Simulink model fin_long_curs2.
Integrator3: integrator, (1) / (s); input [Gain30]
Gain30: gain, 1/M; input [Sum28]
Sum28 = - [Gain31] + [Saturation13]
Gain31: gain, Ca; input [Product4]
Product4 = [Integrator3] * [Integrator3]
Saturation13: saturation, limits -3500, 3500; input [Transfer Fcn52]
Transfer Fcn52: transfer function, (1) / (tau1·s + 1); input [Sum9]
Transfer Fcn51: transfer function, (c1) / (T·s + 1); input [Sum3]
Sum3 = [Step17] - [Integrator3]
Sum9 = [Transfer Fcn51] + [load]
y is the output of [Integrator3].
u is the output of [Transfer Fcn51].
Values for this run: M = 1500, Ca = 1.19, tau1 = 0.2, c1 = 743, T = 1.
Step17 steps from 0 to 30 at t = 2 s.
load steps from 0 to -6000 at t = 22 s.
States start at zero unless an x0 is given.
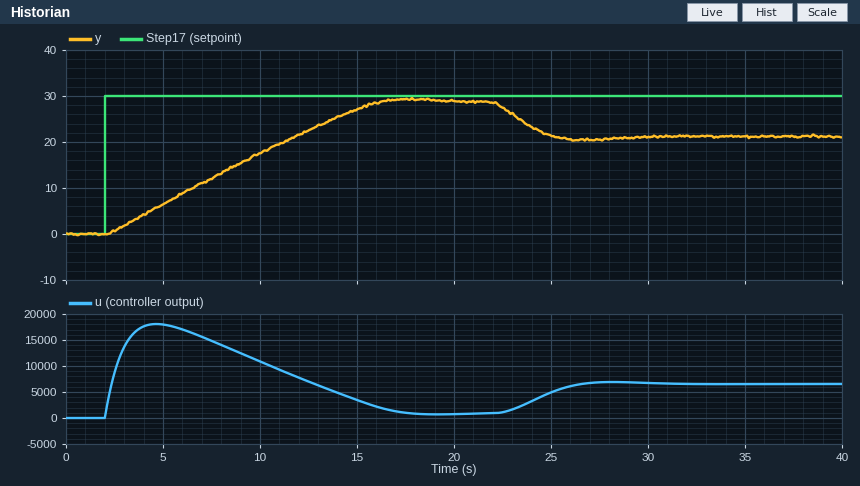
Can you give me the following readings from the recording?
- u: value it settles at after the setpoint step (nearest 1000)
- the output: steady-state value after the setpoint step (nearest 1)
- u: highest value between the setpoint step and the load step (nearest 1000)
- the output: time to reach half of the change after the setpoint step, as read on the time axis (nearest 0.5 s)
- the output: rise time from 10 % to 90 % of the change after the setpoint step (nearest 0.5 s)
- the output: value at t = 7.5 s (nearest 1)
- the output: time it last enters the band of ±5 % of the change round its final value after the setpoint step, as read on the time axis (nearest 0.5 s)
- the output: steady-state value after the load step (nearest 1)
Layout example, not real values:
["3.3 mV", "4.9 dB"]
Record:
["1000", "29", "18000", "8.5 s", "11.0 s", "12", "15.0 s", "21"]
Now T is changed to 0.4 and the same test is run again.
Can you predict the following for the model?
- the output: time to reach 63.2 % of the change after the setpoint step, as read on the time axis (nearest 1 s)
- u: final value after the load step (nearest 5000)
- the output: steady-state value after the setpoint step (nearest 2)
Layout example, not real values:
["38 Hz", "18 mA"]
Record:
["10 s", "5000", "28"]
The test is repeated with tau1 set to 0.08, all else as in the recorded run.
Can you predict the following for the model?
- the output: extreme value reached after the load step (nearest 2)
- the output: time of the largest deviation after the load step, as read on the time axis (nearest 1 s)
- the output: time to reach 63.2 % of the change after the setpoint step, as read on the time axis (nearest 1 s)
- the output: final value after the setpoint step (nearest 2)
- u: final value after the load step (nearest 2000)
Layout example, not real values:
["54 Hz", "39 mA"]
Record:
["20", "27 s", "10 s", "28", "6000"]
